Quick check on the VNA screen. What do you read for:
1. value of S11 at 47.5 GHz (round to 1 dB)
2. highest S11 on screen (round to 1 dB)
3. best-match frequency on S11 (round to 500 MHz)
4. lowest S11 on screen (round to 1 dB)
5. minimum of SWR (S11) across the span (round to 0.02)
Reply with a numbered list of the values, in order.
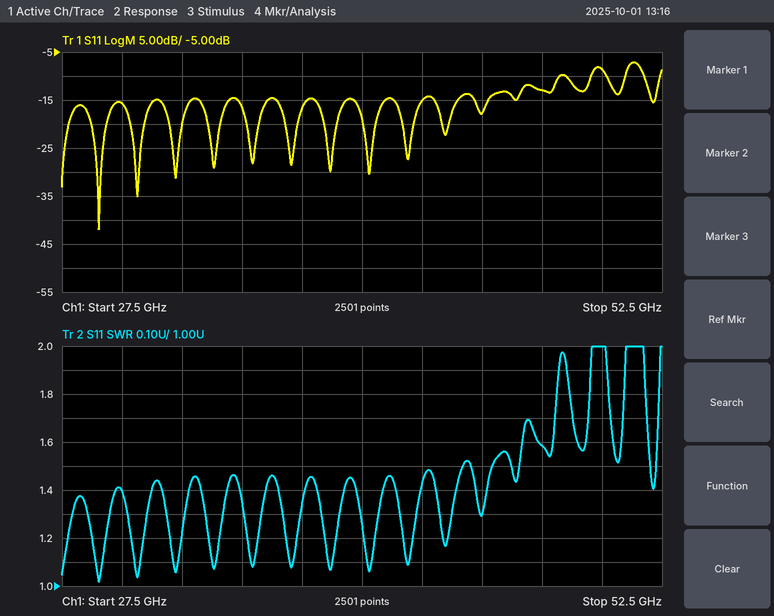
1. -13 dB
2. -7 dB
3. 29.0 GHz
4. -42 dB
5. 1.02
